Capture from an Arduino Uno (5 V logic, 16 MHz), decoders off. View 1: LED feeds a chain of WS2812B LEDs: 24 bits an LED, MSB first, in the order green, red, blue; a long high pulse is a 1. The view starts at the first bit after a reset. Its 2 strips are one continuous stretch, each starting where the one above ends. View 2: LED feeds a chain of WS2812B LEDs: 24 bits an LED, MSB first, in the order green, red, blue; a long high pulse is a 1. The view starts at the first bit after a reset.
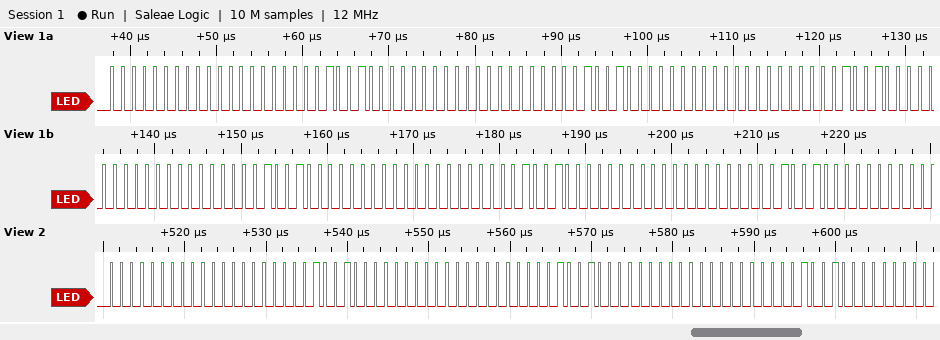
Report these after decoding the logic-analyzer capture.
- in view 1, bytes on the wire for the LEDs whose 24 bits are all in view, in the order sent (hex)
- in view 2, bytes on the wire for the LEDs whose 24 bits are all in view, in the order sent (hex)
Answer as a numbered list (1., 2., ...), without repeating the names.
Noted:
1. 00 00 09 00 00 09 00 00 09 00 00 09 00 00 09 00 00 09
2. 00 00 09 00 00 09 00 00 09
